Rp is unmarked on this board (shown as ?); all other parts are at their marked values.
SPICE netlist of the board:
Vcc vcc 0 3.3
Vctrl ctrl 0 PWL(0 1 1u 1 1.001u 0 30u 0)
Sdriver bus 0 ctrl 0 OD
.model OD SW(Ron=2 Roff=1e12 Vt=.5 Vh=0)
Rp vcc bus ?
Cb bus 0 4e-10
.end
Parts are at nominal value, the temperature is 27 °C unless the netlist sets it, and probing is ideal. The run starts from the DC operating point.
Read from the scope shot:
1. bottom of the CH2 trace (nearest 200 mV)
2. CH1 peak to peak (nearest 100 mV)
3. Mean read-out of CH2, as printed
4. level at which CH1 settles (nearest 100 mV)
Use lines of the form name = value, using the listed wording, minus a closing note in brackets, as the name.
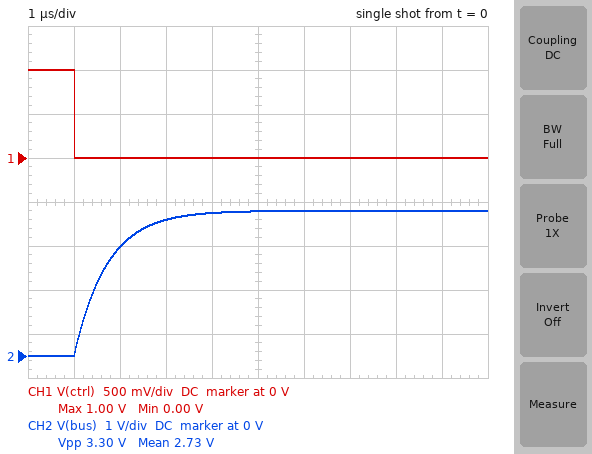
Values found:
bottom of the CH2 trace = 0 V
CH1 peak to peak = 1.0 V
Mean read-out of CH2, as printed = 2.73 V
level at which CH1 settles = 0 V
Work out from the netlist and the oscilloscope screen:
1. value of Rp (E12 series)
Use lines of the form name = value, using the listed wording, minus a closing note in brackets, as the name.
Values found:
value of Rp = 1.8 kΩ
